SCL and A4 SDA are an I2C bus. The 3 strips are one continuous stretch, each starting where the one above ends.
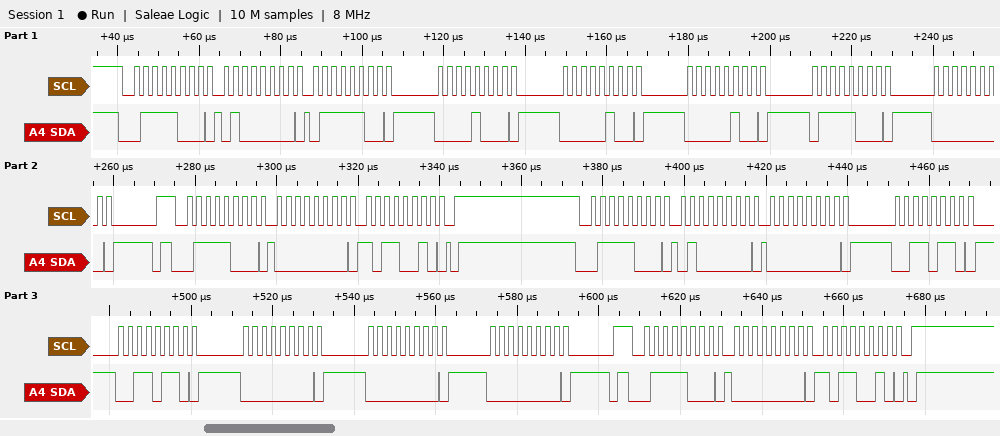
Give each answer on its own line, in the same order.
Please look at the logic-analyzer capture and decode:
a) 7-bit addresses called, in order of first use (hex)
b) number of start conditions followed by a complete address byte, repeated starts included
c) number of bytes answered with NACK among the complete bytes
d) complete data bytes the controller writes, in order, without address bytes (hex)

0x3C
4
0
40 7C 08 04 04 78 00 00 B2 40 00 36 36 00 00 00 00 B2
